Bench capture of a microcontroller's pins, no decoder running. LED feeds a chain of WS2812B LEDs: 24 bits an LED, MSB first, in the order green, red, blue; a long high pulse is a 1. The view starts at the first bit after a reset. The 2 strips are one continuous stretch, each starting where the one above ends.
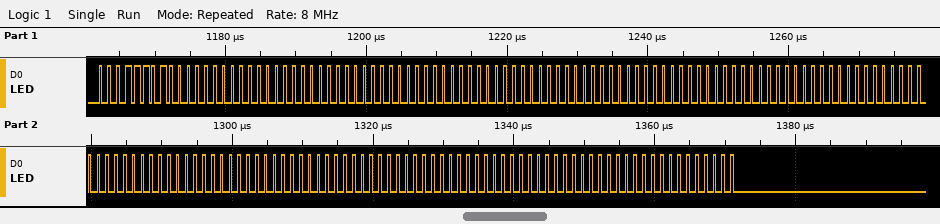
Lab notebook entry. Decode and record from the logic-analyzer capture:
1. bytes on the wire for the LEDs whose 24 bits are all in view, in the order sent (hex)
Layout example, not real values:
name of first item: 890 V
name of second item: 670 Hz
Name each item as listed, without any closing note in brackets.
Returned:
bytes on the wire for the LEDs whose 24 bits are all in view, in the order sent: 1D 00 00 00 00 00 00 00 00 00 00 00 00 00 00 00 00 00 00 00 00
